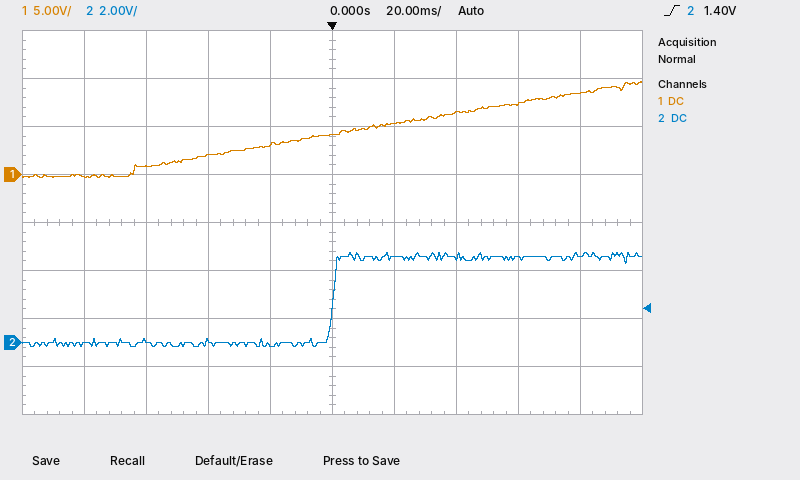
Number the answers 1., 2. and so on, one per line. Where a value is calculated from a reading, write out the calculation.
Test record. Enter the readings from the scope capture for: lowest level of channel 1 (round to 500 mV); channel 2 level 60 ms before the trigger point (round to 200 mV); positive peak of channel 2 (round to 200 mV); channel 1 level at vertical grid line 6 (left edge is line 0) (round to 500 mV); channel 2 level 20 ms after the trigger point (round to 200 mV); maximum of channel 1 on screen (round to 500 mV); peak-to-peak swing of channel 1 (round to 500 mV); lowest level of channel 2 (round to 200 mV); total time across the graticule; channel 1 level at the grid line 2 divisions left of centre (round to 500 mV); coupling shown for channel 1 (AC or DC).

1. -500 mV
2. 0.0 V
3. 3.8 V
4. 5.5 V
5. 3.6 V
6. 9.5 V
7. 9.5 V − (-500 mV) = 10.0 V
8. -200 mV
9. 200 ms
10. 2.0 V
11. DC
